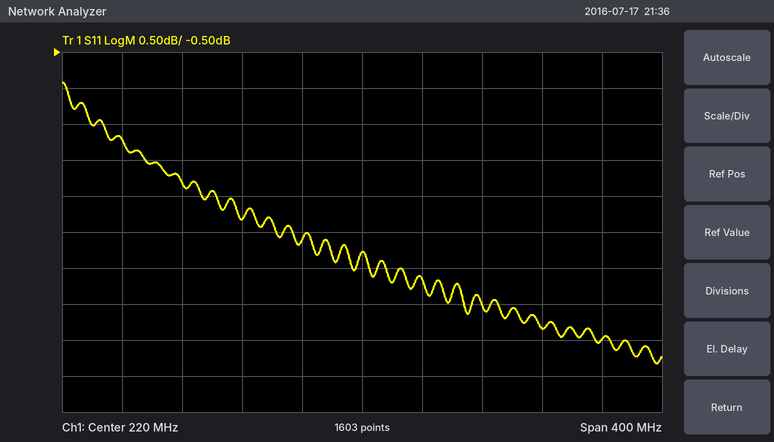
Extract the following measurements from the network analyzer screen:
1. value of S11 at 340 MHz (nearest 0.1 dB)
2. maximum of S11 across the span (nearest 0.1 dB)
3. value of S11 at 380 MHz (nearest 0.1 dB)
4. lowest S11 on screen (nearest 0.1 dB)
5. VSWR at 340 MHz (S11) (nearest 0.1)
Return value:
-4.3 dB
-0.9 dB
-4.5 dB
-4.8 dB
4.1
